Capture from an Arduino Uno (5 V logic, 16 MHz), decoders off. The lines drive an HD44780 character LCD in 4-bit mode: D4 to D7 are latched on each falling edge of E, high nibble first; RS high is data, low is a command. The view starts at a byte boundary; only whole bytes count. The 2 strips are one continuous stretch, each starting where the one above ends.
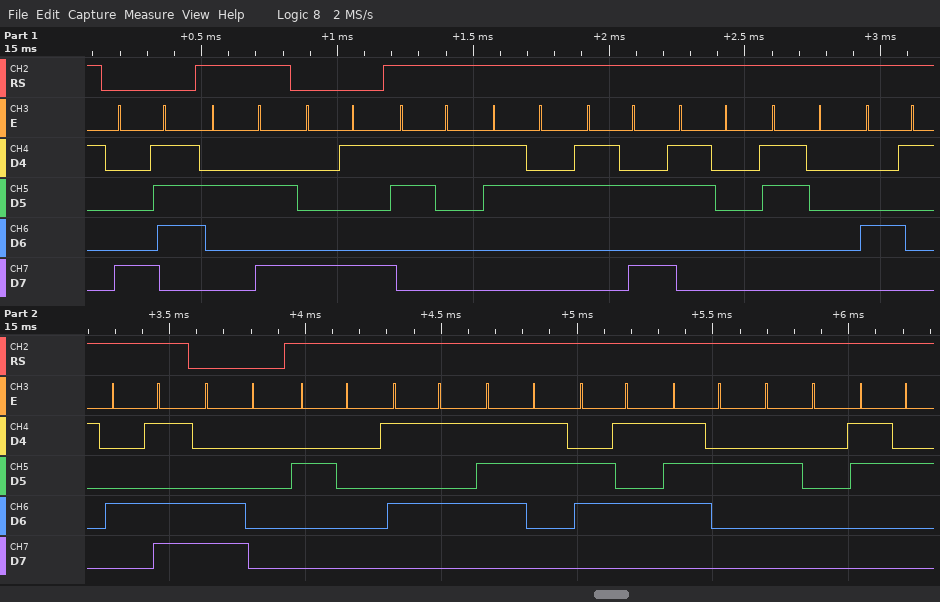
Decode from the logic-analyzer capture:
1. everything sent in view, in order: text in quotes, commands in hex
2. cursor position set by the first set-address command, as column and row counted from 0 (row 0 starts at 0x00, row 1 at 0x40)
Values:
0x87 "*" 0x89 "12:00AM" 0xC0 " User 2"
column 7, row 0
